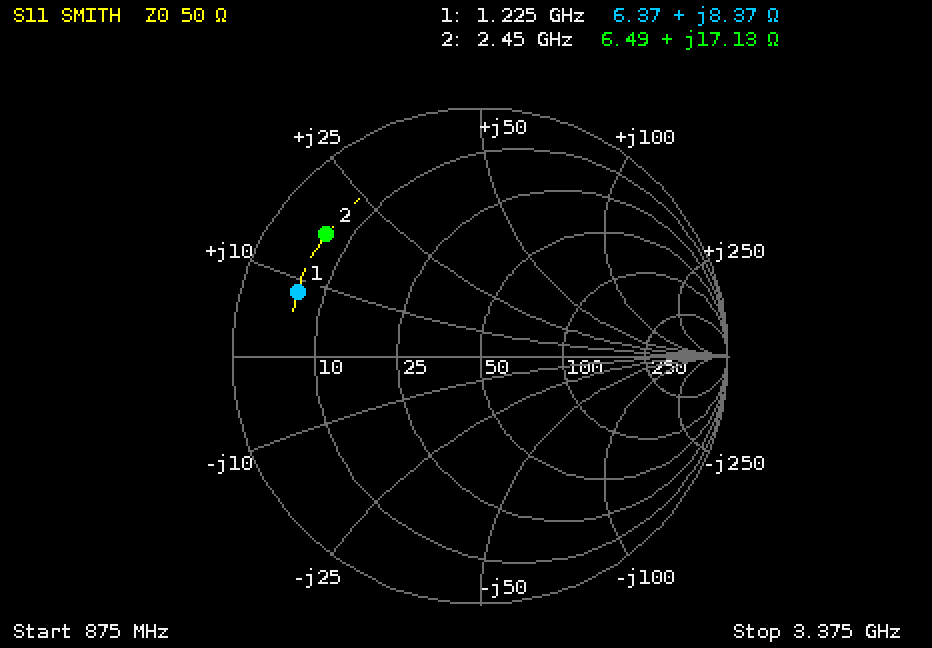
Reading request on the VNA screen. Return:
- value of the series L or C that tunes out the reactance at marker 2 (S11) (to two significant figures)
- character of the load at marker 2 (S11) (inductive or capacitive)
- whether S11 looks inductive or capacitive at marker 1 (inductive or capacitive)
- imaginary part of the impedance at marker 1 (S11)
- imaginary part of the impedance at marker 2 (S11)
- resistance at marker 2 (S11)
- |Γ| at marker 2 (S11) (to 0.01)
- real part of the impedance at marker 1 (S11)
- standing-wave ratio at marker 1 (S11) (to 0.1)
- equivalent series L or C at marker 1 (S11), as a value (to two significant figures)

3.8 pF
inductive
inductive
+8.37 Ω
+17.13 Ω
6.49 Ω
0.79
6.37 Ω
8.1
1.1 nH
